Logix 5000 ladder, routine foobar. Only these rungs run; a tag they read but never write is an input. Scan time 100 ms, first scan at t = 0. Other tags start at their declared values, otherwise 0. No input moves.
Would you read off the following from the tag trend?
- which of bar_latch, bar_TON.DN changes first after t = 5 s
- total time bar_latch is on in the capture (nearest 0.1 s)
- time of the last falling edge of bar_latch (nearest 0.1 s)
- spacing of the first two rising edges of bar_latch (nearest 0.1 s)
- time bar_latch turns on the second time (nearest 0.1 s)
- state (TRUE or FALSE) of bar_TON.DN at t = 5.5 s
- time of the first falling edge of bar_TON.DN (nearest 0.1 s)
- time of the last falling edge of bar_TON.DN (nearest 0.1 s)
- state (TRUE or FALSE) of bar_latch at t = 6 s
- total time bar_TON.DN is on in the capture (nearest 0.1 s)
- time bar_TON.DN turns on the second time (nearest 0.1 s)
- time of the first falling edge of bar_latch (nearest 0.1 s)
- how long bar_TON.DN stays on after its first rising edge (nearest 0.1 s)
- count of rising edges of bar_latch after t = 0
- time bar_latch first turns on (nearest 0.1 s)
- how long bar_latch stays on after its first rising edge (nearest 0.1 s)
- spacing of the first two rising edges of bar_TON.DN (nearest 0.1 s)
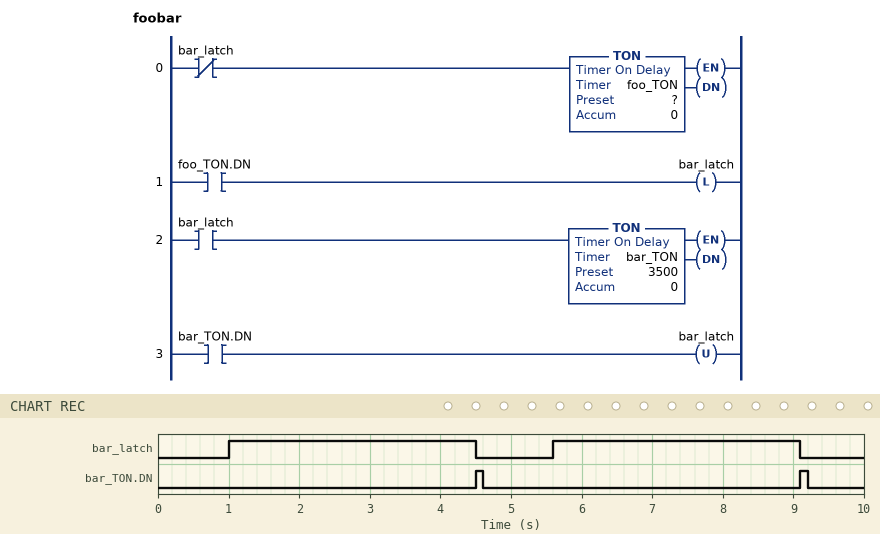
bar_latch
7.0 s
9.1 s
4.6 s
5.6 s
FALSE
4.6 s
9.2 s
TRUE
0.2 s
9.1 s
4.5 s
0.1 s
2
1.0 s
3.5 s
4.6 s
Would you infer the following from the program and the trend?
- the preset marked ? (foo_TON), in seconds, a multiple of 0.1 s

1.0 s
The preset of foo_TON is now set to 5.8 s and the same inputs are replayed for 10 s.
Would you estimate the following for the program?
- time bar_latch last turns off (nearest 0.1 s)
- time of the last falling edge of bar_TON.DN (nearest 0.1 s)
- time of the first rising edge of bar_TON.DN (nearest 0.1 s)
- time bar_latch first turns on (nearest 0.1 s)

9.3 s
9.4 s
9.3 s
5.8 s
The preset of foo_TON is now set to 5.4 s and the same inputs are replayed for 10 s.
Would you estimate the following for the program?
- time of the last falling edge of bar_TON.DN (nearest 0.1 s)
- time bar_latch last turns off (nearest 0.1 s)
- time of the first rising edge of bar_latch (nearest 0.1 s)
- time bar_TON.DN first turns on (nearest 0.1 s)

9.0 s
8.9 s
5.4 s
8.9 s
